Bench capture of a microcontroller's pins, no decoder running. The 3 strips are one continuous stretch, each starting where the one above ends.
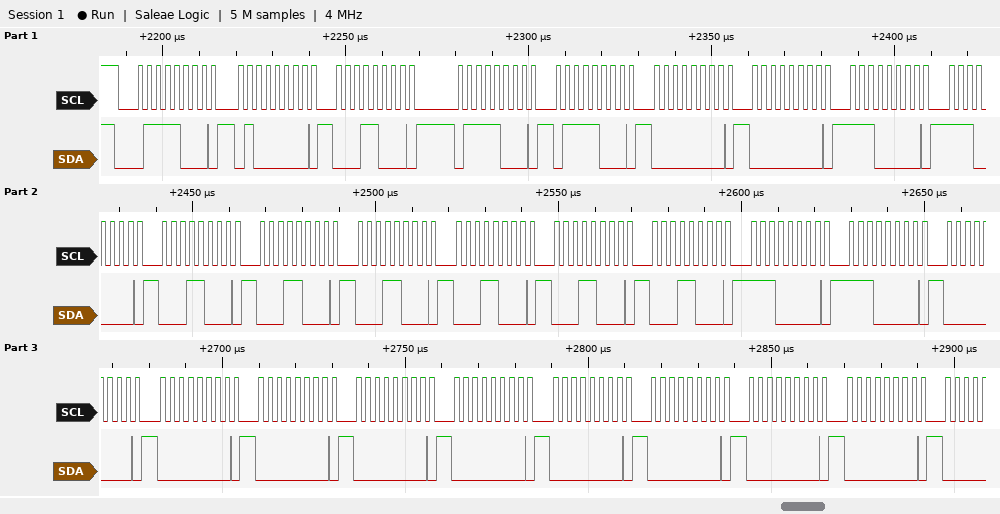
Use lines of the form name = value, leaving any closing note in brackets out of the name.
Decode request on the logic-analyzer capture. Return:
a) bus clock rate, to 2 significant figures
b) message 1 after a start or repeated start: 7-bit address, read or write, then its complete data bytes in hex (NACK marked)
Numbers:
bus clock rate, to 2 significant figures = 400 kHz
message 1 after a start or repeated start: 7-bit address, read or write, then its complete data bytes in hex = 0x3C write: 40 18 78 78 00 00 E0 E0 18 18 18 18 18 18 E0 E0 00 00 00 00 00 00 00 00 00
